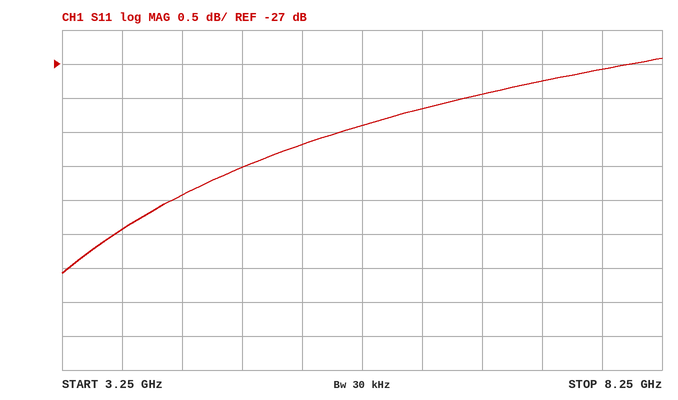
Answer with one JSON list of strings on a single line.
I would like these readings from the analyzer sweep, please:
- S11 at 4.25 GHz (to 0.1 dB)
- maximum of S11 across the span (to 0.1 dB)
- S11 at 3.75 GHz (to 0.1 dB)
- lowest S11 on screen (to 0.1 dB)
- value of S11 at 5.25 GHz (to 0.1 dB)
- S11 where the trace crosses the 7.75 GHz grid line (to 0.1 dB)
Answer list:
["-28.9 dB", "-26.9 dB", "-29.4 dB", "-30.1 dB", "-28.2 dB", "-27.1 dB"]
